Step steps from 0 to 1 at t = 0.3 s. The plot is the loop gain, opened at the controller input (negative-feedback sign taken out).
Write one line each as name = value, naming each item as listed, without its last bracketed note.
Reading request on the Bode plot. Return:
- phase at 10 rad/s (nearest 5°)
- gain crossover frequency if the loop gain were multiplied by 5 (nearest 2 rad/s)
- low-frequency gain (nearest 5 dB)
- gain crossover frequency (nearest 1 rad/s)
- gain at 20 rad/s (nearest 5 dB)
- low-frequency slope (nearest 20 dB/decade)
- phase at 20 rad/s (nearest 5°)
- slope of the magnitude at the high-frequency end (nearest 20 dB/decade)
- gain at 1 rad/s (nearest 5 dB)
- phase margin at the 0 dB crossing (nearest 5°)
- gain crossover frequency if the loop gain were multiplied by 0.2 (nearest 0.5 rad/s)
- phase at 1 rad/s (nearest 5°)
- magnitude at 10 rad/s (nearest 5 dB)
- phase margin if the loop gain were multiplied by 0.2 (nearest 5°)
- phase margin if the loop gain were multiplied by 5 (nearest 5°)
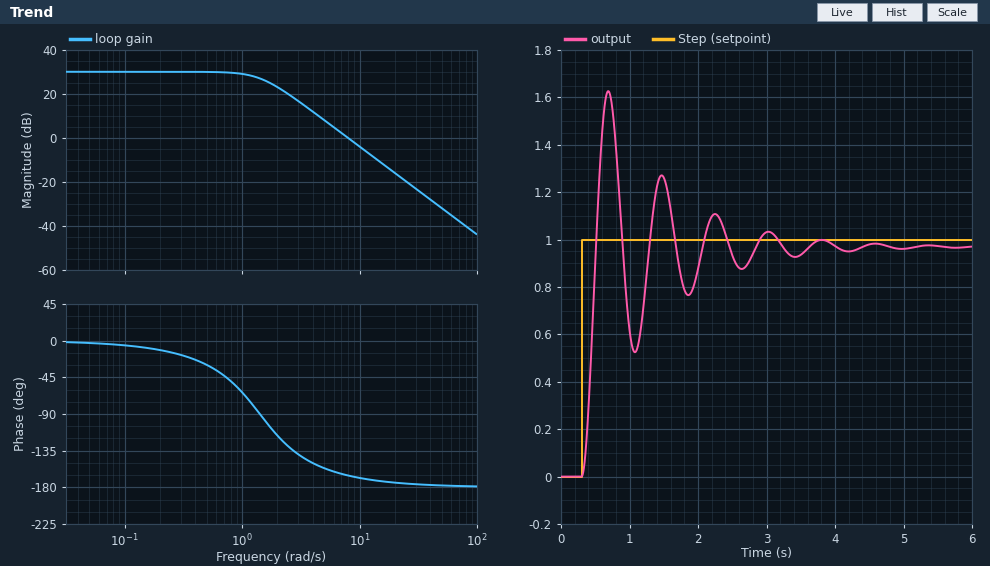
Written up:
phase at 10 rad/s = -170°
gain crossover frequency if the loop gain were multiplied by 5 = 18 rad/s
low-frequency gain = 30 dB
gain crossover frequency = 8 rad/s
gain at 20 rad/s = -15 dB
low-frequency slope = 0 dB/decade
phase at 20 rad/s = -175°
slope of the magnitude at the high-frequency end = -40 dB/decade
gain at 1 rad/s = 30 dB
phase margin at the 0 dB crossing = 15°
gain crossover frequency if the loop gain were multiplied by 0.2 = 3.5 rad/s
phase at 1 rad/s = -65°
magnitude at 10 rad/s = -5 dB
phase margin if the loop gain were multiplied by 0.2 = 35°
phase margin if the loop gain were multiplied by 5 = 5°
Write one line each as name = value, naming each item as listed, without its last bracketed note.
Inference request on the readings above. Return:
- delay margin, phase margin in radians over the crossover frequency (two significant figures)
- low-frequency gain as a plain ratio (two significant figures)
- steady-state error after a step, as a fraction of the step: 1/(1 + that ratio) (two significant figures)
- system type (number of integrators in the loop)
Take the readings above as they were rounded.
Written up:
delay margin, phase margin in radians over the crossover frequency = 0.033 s
low-frequency gain as a plain ratio = 32
steady-state error after a step, as a fraction of the step: 1/(1 + that ratio) = 0.030
system type = 0
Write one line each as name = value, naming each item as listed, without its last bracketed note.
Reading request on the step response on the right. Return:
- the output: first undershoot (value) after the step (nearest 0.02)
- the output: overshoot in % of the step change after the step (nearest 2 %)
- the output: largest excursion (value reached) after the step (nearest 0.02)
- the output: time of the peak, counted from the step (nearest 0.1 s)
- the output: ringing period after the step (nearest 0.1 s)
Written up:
the output: first undershoot (value) after the step = 0.52
the output: overshoot in % of the step change after the step = 68 %
the output: largest excursion (value reached) after the step = 1.62
the output: time of the peak, counted from the step = 0.4 s
the output: ringing period after the step = 0.8 s
